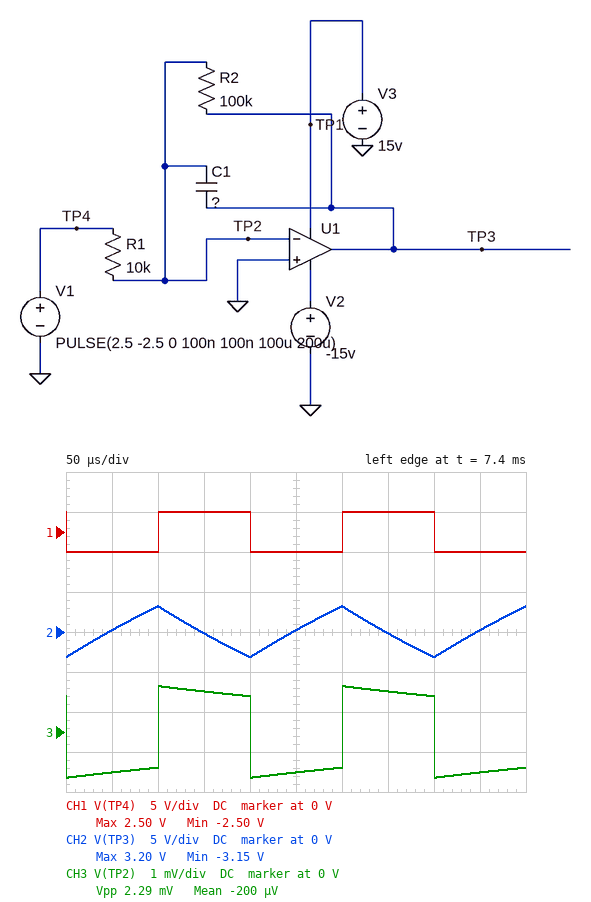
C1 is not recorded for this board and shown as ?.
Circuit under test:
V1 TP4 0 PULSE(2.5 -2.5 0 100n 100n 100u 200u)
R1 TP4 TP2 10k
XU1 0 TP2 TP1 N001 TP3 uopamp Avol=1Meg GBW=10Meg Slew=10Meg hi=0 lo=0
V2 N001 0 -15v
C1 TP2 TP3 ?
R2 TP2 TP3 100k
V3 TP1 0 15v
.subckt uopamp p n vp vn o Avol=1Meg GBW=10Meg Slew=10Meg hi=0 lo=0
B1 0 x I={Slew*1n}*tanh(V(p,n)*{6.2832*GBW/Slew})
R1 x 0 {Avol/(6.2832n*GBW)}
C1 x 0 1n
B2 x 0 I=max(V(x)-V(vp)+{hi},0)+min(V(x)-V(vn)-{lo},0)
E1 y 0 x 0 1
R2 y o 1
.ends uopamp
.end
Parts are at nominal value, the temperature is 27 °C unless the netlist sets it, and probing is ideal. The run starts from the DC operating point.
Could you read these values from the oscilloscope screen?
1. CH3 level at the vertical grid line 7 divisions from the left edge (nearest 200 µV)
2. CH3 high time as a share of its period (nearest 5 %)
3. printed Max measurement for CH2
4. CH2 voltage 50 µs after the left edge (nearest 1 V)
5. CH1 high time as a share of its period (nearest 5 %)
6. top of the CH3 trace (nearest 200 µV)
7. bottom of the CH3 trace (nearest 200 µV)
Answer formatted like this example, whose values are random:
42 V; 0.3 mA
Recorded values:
1.0 mV; 50 %; 3.20 V; 0 V; 50 %; 1.2 mV; -1.2 mV
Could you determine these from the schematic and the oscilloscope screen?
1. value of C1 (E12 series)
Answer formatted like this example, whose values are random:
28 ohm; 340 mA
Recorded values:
3.9 nF
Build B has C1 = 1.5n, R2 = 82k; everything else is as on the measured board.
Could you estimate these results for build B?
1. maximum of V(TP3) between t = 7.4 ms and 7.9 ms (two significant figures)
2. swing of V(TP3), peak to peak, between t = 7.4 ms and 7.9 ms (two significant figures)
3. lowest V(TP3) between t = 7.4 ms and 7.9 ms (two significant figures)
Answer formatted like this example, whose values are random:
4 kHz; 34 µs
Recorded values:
7.9 V; 16 V; -7.9 V
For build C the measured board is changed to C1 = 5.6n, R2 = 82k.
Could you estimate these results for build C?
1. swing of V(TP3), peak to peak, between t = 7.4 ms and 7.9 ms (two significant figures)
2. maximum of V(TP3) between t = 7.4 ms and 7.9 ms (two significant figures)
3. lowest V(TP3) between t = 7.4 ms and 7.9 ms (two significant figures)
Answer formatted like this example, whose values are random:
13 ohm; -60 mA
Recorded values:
4.4 V; 2.2 V; -2.2 V
